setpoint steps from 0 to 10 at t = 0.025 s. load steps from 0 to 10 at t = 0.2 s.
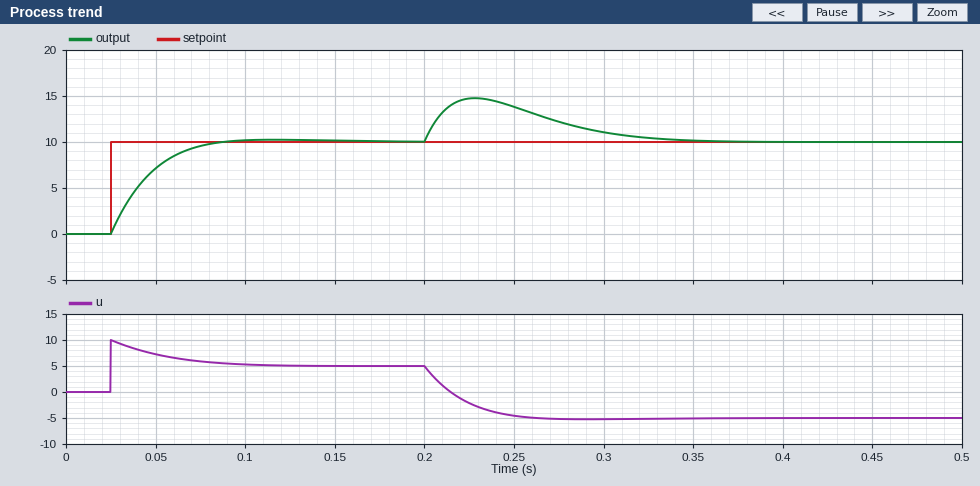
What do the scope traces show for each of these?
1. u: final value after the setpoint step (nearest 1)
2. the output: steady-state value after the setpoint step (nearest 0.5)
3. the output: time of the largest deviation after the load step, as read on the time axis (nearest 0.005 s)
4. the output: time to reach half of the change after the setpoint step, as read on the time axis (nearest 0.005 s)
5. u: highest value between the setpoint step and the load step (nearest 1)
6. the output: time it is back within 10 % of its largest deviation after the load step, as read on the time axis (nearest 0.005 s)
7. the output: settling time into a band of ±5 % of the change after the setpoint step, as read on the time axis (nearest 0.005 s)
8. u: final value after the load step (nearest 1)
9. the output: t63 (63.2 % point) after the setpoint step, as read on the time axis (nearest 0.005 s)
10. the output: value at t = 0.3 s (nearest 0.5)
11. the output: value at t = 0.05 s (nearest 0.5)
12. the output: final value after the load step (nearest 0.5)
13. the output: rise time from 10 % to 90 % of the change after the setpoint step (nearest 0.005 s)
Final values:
5
10.0
0.230 s
0.040 s
10
0.325 s
0.075 s
-5
0.045 s
11.0
7.0
10.0
0.040 s
